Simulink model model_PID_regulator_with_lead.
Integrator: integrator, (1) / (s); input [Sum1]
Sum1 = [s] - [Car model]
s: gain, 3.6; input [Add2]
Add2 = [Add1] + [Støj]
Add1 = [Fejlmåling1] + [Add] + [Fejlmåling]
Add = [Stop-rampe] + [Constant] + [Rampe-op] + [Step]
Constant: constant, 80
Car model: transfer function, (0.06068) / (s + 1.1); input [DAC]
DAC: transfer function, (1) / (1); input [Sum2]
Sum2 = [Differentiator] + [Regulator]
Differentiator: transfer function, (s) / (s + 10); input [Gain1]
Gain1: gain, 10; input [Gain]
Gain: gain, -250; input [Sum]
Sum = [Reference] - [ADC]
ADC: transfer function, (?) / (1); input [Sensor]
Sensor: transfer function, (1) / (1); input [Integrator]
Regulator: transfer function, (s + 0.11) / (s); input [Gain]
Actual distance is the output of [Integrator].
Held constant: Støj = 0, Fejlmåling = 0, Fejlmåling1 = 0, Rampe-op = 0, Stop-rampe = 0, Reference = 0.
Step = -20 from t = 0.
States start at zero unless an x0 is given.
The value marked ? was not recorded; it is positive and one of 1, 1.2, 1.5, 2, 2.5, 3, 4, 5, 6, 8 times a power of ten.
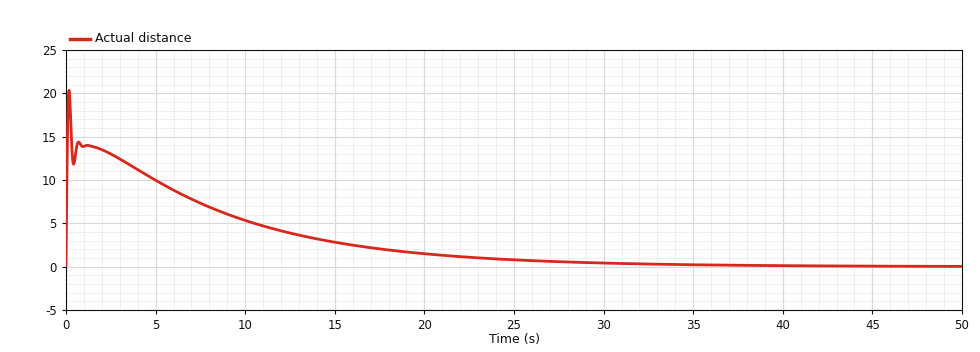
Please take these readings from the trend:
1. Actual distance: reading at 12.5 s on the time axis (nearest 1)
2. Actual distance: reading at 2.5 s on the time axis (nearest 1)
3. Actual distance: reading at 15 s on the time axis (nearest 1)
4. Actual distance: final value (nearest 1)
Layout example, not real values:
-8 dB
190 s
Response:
4
13
3
0
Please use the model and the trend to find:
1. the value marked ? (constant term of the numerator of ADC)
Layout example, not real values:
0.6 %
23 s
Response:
1
